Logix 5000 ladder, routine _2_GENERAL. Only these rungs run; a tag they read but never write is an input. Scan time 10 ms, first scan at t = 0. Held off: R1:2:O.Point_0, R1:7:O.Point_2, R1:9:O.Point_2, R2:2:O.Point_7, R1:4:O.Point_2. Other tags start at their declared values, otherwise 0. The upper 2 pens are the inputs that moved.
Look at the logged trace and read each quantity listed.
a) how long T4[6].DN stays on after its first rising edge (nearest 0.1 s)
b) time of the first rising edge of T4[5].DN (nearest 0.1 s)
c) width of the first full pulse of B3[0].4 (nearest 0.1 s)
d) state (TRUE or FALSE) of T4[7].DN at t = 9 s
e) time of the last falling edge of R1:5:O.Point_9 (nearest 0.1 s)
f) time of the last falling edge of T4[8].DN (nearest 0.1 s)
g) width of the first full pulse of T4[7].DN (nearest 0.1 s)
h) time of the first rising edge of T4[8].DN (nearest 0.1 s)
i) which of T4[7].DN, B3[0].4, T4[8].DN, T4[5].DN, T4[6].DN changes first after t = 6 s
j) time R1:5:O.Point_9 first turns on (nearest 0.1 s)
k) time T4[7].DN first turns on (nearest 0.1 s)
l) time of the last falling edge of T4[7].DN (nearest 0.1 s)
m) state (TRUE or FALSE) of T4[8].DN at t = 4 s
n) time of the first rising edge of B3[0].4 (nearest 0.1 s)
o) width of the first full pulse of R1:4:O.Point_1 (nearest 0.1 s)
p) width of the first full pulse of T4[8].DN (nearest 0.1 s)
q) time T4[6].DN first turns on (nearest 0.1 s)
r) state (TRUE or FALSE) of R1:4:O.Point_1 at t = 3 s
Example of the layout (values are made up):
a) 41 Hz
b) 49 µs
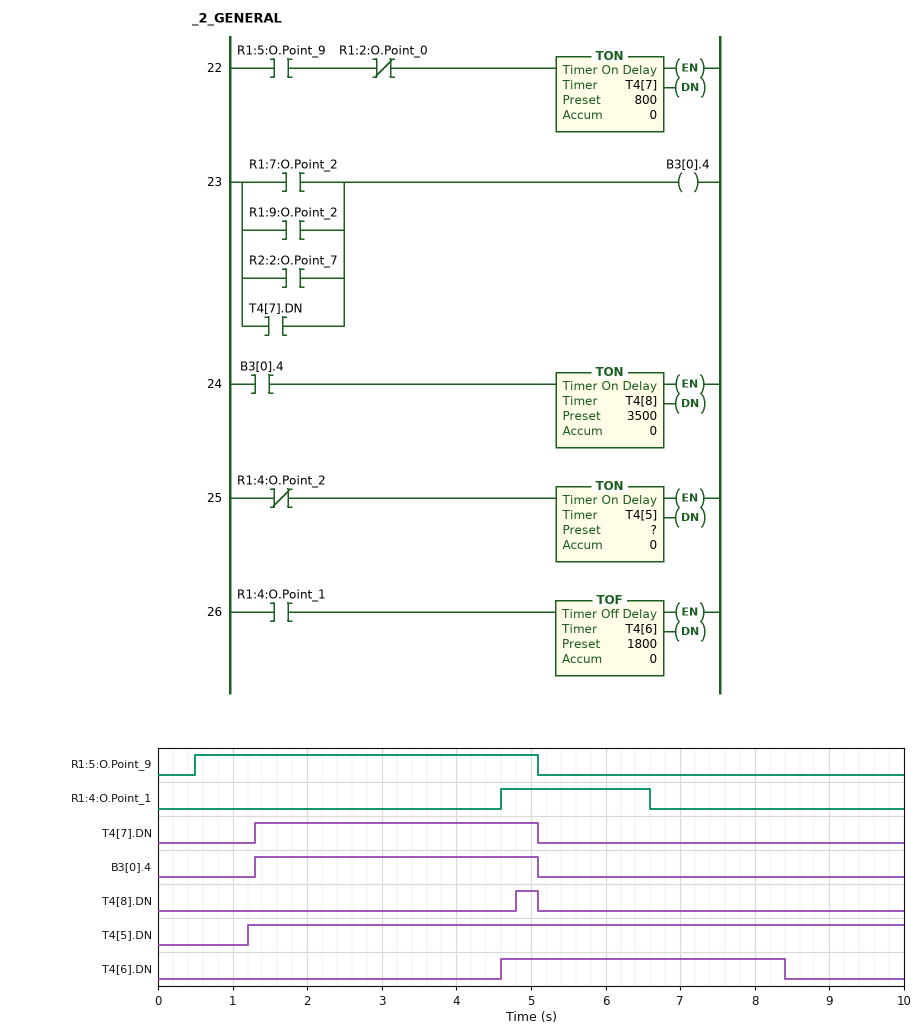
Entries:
a) 3.8 s
b) 1.2 s
c) 3.8 s
d) FALSE
e) 5.1 s
f) 5.1 s
g) 3.8 s
h) 4.8 s
i) T4[6].DN
j) 0.5 s
k) 1.3 s
l) 5.1 s
m) FALSE
n) 1.3 s
o) 2.0 s
p) 0.3 s
q) 4.6 s
r) FALSE
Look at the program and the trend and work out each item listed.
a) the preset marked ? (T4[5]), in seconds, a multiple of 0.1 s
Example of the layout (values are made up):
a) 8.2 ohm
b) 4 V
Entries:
a) 1.2 s
